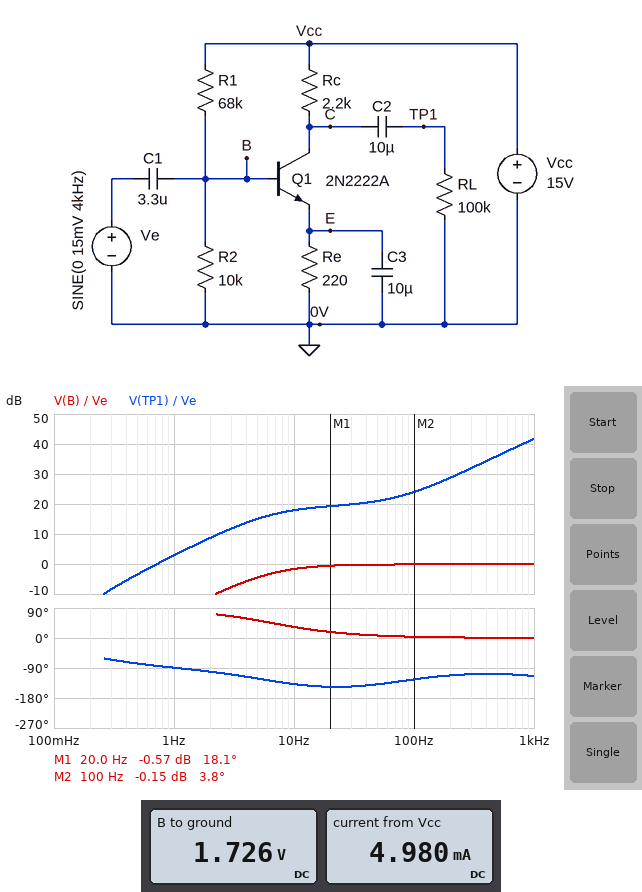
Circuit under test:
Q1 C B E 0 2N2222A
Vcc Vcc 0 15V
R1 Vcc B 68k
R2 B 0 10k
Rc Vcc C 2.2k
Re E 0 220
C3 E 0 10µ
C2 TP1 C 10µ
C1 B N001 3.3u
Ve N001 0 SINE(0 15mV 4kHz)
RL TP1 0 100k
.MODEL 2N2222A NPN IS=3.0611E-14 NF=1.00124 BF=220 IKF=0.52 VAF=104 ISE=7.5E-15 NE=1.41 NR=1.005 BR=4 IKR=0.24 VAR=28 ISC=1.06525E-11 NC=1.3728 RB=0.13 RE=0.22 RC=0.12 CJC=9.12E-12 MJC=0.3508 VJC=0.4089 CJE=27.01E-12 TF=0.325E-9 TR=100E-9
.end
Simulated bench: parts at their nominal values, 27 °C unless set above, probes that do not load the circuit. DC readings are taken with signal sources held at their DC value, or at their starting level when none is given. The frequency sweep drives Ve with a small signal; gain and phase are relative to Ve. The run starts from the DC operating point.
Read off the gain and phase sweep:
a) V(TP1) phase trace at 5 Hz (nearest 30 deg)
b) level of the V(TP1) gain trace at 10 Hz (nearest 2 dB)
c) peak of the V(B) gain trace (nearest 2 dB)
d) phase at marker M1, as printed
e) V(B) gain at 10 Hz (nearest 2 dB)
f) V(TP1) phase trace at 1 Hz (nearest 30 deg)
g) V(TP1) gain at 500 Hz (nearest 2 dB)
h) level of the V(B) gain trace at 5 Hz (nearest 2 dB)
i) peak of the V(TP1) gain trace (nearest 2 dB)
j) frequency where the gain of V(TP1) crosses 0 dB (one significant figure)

-120 deg
18 dB
0 dB
18.1 deg
-2 dB
-90 deg
36 dB
-4 dB
42 dB
700 mHz
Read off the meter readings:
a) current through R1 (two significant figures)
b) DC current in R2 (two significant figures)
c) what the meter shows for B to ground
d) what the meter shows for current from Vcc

200 µA
170 µA
1.726 V
4.980 mA
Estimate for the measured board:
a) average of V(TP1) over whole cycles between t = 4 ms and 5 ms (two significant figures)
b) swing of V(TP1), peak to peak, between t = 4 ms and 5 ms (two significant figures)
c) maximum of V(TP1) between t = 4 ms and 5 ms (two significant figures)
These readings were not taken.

430 mV
7.5 V
4.1 V
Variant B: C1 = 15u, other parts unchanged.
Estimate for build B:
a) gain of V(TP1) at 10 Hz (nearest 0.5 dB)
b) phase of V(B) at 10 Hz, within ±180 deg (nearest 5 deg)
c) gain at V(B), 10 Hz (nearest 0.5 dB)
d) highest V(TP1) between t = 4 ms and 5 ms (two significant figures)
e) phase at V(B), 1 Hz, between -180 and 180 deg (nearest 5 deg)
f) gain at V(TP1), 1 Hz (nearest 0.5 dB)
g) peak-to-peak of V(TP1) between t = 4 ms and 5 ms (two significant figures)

19.5 dB
10 deg
0 dB
4.0 V
55 deg
14.5 dB
7.3 V
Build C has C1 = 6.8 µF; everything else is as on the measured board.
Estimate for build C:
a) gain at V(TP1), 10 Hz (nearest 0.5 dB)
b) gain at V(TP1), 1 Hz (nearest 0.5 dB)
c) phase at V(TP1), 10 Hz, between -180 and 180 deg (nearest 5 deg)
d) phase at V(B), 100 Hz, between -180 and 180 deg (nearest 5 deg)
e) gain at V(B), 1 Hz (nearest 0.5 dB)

19.0 dB
9.0 dB
-155 deg
0 deg
-10.5 dB
